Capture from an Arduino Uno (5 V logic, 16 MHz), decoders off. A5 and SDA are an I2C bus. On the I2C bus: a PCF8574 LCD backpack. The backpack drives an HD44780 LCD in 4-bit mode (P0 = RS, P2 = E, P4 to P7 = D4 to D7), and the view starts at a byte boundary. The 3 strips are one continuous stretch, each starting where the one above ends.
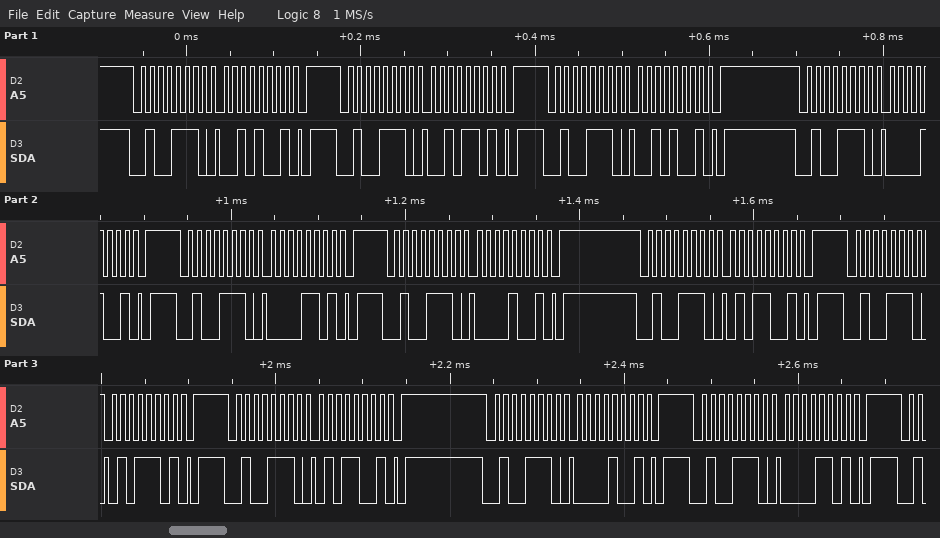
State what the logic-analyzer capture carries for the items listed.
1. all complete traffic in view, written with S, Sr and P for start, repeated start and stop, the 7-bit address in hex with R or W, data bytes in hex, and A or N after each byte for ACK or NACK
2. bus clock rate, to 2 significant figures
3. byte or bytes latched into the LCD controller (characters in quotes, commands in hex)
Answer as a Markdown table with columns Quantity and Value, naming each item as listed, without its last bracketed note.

| Quantity | Value |
|---|---|
| all complete traffic in view, written with S, Sr and P for start, repeated start and stop, the 7-bit address in hex with R or W, data bytes in hex, and A or N after each byte for ACK or NACK | S 27W A 29 A P S 27W A 2D A P S 27W A 29 A P S 27W A 09 A P S 27W A 0D A P S 27W A 09 A P S 27W A 59 A P S 27W A 5D A P S 27W A 59 A P S 27W A 09 A P S 27W A 0D A P |
| bus clock rate, to 2 significant figures | 100 kHz |
| byte or bytes latched into the LCD controller | ' ' |
